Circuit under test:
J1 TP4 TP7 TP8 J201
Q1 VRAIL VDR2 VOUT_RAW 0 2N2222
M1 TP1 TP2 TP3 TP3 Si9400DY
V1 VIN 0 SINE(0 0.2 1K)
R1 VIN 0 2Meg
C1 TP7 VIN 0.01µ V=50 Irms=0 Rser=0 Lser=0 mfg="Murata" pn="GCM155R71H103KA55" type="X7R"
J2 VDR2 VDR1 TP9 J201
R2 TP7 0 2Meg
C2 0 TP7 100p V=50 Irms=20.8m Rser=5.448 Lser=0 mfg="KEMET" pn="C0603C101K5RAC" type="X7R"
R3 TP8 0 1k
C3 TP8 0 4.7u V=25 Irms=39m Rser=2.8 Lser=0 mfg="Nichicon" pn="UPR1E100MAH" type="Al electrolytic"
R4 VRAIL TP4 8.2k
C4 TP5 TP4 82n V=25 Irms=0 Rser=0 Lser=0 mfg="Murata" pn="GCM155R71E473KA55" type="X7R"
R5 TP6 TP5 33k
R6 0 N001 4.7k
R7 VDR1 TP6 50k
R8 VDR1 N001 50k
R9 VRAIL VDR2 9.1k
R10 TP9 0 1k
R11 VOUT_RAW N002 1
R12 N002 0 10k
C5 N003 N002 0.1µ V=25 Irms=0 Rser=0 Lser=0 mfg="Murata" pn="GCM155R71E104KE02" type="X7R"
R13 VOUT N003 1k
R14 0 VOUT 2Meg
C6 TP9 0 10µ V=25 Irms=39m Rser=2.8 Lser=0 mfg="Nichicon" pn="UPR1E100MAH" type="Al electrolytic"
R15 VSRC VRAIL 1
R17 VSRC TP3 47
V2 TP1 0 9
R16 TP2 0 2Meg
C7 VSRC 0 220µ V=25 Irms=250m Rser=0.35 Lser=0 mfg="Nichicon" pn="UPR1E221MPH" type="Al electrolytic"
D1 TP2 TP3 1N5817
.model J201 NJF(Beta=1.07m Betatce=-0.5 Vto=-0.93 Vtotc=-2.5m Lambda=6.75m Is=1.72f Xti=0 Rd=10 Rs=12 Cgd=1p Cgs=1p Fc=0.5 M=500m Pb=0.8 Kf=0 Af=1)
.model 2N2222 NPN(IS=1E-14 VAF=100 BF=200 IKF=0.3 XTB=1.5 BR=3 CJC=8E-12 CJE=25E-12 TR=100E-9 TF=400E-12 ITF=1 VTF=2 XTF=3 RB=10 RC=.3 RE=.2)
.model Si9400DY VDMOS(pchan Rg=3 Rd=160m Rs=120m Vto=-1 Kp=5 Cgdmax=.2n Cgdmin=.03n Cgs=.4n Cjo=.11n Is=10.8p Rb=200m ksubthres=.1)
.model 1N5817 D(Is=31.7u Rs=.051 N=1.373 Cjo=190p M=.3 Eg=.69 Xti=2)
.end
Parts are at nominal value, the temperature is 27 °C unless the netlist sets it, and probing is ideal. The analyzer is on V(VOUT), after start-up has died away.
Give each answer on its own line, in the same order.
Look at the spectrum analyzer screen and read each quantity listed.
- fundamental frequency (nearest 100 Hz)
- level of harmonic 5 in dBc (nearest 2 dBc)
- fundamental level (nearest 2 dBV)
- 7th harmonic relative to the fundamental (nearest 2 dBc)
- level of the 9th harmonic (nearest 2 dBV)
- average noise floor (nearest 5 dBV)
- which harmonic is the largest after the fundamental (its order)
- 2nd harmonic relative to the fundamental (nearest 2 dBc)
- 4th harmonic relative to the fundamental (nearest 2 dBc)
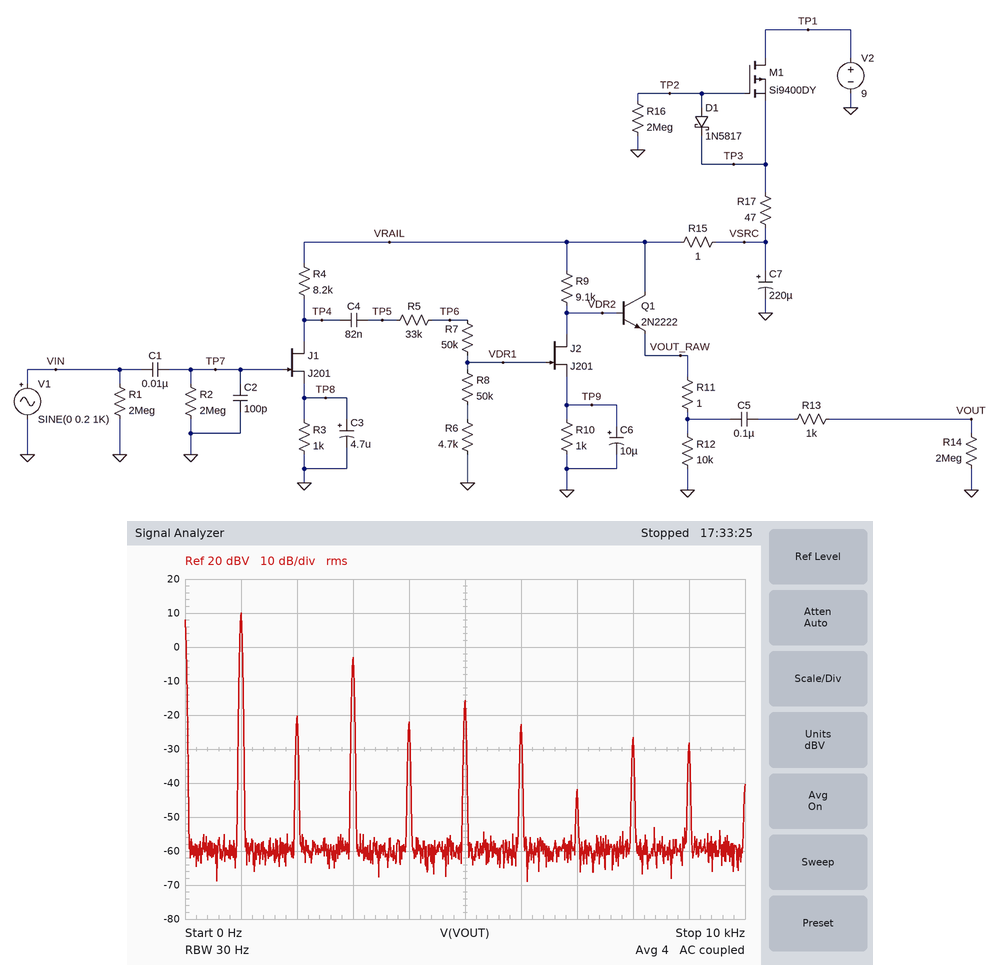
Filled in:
1.0 kHz
-26 dBc
10 dBV
-52 dBc
-28 dBV
-60 dBV
3
-30 dBc
-32 dBc
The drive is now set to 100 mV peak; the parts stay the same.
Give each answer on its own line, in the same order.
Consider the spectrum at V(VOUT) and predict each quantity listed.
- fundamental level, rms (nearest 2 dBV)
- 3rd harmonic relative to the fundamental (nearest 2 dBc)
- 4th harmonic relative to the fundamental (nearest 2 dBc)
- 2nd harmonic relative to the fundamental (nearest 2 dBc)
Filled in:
8 dBV
-30 dBc
-40 dBc
-20 dBc
